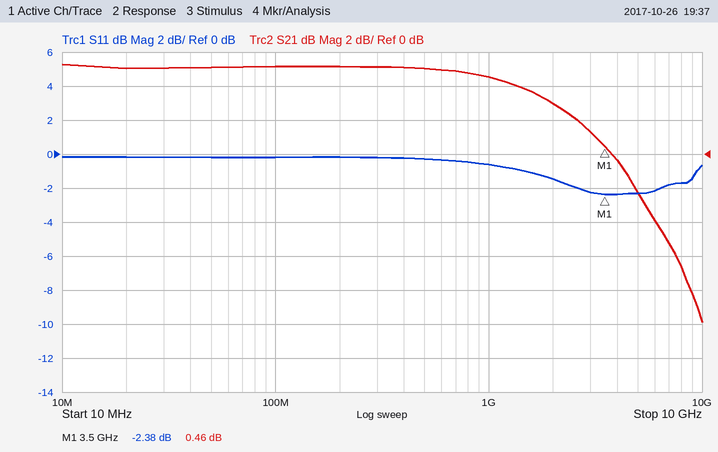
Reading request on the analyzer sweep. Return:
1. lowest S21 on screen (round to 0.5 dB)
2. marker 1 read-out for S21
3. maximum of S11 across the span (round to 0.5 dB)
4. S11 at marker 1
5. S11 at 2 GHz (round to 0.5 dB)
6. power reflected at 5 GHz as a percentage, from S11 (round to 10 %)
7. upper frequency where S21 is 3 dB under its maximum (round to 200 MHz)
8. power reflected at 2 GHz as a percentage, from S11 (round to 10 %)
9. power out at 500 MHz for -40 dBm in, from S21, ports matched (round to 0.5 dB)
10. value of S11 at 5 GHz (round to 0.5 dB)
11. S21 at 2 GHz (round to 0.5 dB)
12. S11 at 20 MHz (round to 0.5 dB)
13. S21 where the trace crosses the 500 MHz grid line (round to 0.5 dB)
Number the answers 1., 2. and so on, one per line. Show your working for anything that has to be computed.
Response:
1. -10.0 dB
2. 0.46 dB
3. 0.0 dB
4. -2.38 dB
5. -1.5 dB
6. 10^(-2.5/10) ≈ 56.2 %, so 60 % to the nearest 10 %
7. 2.4 GHz
8. 10^(-1.5/10) ≈ 70.8 %, so 70 % to the nearest 10 %
9. -40 dBm + (5.0 dB) = -35.0 dBm
10. -2.5 dB
11. 3.0 dB
12. 0.0 dB
13. 5.0 dB
